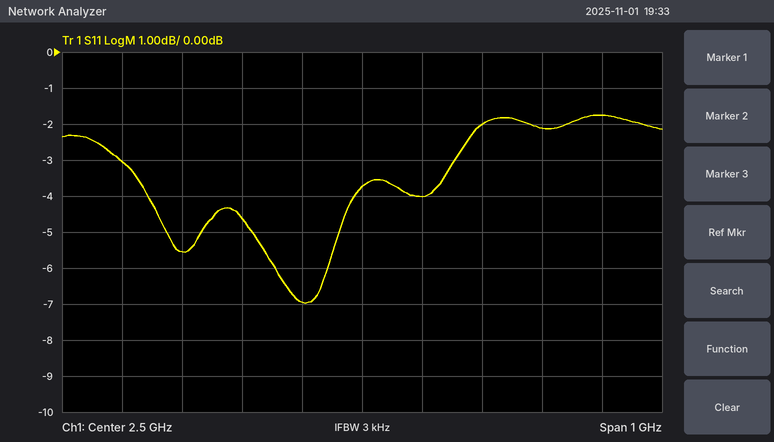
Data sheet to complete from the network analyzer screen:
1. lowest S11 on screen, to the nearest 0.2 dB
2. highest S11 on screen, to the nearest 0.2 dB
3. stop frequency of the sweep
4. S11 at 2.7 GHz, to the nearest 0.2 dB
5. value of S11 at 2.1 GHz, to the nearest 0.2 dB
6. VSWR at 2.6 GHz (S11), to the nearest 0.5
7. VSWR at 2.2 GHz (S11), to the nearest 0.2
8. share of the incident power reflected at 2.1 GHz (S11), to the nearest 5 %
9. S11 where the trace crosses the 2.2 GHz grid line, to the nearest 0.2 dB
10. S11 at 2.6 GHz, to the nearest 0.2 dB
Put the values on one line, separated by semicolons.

-7.0 dB; -1.8 dB; 3 GHz; -2.0 dB; -3.0 dB; 4.5; 3.2; 50 %; -5.6 dB; -4.0 dB
